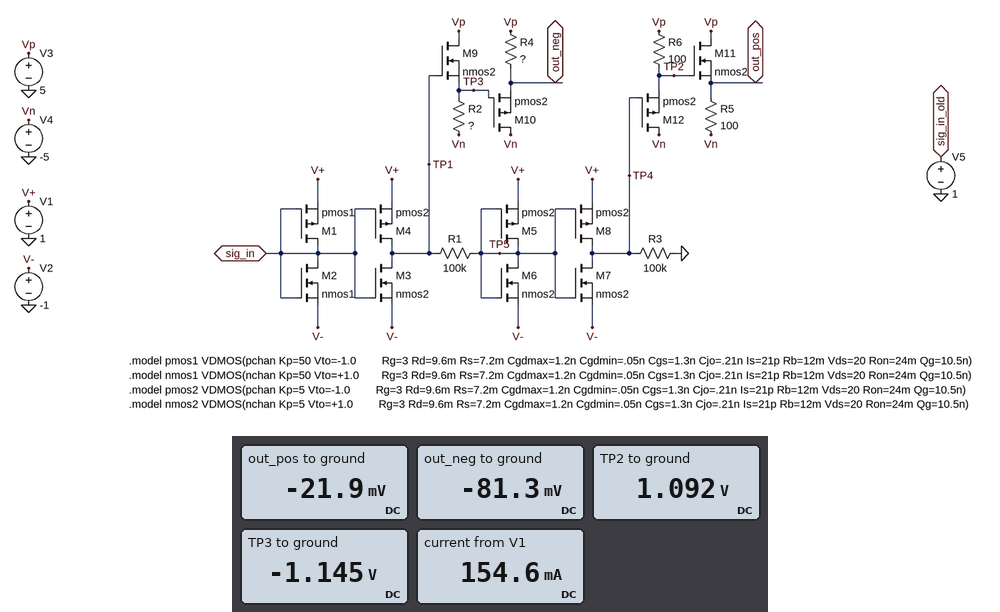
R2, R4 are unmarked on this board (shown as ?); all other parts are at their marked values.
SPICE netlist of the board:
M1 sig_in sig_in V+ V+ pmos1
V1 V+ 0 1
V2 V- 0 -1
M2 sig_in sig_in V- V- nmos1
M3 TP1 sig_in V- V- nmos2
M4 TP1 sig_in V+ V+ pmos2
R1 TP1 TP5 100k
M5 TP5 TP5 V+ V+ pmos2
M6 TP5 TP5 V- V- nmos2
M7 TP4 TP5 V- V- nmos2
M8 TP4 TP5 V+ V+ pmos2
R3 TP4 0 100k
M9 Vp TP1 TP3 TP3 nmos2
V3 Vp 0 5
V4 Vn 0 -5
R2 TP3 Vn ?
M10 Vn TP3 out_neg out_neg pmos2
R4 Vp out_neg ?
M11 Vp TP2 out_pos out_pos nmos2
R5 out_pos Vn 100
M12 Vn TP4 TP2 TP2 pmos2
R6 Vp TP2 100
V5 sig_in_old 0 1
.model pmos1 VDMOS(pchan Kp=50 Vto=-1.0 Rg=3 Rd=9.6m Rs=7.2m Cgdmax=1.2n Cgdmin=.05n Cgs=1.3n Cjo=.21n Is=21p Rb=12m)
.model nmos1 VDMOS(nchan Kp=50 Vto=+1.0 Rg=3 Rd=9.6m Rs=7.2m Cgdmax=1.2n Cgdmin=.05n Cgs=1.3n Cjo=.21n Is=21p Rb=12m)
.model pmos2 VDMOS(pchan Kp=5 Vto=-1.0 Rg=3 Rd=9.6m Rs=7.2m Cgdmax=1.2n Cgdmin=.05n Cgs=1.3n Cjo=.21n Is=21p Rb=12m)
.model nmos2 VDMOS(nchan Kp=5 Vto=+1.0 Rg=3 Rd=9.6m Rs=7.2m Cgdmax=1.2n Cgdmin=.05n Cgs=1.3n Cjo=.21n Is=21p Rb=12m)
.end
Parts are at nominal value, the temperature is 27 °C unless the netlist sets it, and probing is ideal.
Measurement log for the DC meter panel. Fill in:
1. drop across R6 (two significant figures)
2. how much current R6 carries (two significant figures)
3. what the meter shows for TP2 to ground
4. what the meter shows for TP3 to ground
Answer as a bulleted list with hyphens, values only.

- 3.9 V
- 39 mA
- 1.092 V
- -1.145 V
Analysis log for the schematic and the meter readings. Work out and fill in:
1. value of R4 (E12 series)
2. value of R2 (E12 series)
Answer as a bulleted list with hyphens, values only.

- 180 Ω
- 56 Ω
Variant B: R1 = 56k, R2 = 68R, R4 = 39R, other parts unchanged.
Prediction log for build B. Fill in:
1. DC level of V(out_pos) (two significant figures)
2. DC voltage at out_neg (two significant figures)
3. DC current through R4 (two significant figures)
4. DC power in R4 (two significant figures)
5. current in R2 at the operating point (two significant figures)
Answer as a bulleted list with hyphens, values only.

- -22 mV
- 88 mV
- 130 mA
- 620 mW
- 57 mA
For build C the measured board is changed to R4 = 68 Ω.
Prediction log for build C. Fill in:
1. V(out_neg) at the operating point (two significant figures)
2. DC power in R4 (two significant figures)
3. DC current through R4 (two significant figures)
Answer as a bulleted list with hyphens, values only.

- 6.7 mV
- 370 mW
- 73 mA
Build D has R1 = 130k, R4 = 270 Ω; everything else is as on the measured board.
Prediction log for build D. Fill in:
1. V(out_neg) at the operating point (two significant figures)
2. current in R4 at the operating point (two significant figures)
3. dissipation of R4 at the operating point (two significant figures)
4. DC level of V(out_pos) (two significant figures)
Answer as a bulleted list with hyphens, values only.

- -110 mV
- 19 mA
- 97 mW
- -22 mV
